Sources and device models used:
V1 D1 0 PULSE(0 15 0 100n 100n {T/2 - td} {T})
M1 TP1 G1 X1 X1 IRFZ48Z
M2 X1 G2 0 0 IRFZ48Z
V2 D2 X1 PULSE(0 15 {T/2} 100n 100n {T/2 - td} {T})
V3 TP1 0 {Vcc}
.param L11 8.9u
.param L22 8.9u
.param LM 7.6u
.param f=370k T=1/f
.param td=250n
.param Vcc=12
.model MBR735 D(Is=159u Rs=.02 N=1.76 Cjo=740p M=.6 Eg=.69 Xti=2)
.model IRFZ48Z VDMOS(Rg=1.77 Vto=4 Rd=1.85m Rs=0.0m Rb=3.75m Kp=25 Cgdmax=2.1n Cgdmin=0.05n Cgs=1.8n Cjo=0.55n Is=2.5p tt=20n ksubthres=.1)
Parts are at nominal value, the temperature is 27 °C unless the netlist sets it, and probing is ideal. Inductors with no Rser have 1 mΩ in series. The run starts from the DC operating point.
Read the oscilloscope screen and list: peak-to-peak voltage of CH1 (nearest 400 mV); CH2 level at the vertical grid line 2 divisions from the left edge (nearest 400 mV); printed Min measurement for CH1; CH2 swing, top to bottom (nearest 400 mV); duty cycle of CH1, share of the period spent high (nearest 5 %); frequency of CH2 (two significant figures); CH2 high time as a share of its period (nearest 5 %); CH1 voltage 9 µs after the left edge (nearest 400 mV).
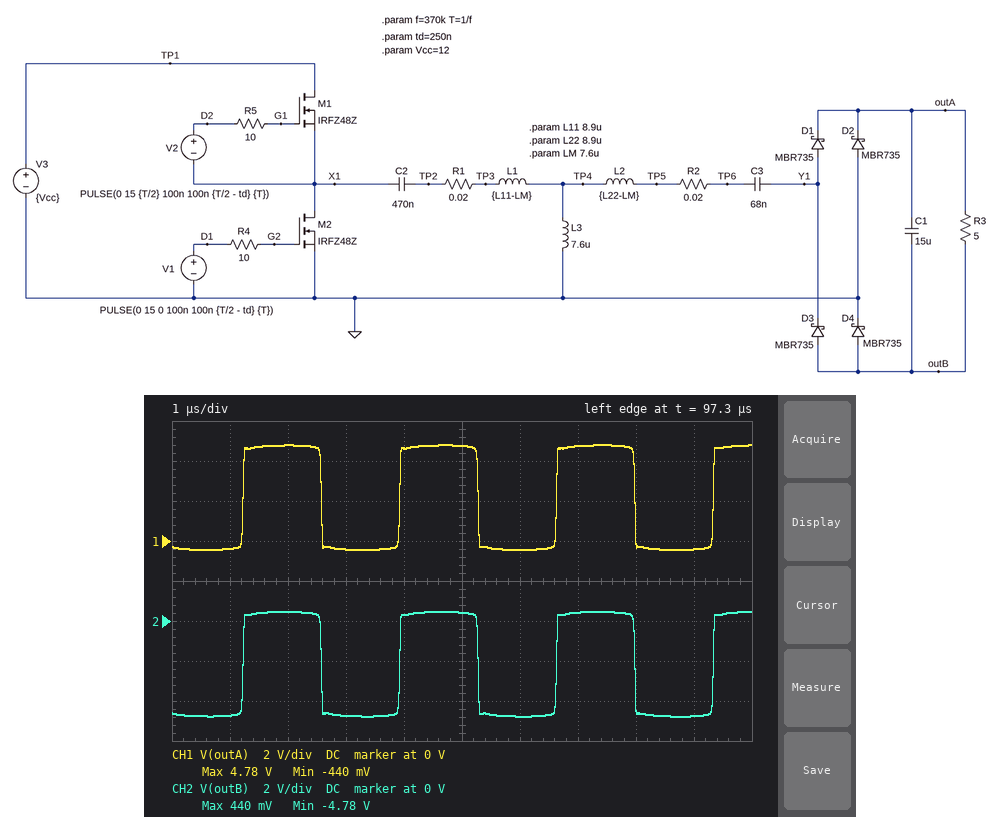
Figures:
5.2 V
400 mV
-440 mV
5.2 V
50 %
370 kHz
50 %
-400 mV
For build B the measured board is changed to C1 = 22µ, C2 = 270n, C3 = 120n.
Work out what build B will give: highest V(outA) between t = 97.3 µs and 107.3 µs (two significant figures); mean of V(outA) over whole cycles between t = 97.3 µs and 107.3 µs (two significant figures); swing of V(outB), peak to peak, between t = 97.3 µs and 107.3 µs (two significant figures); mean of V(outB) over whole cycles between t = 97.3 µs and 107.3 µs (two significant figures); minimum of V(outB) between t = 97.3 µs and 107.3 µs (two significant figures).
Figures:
5.1 V
2.3 V
5.5 V
-2.3 V
-5.1 V
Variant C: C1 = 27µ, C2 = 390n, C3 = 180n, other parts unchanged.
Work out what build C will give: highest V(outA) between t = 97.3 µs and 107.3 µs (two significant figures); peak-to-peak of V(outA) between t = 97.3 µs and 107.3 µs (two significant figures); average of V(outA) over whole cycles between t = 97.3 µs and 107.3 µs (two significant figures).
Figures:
4.0 V
4.4 V
1.7 V
